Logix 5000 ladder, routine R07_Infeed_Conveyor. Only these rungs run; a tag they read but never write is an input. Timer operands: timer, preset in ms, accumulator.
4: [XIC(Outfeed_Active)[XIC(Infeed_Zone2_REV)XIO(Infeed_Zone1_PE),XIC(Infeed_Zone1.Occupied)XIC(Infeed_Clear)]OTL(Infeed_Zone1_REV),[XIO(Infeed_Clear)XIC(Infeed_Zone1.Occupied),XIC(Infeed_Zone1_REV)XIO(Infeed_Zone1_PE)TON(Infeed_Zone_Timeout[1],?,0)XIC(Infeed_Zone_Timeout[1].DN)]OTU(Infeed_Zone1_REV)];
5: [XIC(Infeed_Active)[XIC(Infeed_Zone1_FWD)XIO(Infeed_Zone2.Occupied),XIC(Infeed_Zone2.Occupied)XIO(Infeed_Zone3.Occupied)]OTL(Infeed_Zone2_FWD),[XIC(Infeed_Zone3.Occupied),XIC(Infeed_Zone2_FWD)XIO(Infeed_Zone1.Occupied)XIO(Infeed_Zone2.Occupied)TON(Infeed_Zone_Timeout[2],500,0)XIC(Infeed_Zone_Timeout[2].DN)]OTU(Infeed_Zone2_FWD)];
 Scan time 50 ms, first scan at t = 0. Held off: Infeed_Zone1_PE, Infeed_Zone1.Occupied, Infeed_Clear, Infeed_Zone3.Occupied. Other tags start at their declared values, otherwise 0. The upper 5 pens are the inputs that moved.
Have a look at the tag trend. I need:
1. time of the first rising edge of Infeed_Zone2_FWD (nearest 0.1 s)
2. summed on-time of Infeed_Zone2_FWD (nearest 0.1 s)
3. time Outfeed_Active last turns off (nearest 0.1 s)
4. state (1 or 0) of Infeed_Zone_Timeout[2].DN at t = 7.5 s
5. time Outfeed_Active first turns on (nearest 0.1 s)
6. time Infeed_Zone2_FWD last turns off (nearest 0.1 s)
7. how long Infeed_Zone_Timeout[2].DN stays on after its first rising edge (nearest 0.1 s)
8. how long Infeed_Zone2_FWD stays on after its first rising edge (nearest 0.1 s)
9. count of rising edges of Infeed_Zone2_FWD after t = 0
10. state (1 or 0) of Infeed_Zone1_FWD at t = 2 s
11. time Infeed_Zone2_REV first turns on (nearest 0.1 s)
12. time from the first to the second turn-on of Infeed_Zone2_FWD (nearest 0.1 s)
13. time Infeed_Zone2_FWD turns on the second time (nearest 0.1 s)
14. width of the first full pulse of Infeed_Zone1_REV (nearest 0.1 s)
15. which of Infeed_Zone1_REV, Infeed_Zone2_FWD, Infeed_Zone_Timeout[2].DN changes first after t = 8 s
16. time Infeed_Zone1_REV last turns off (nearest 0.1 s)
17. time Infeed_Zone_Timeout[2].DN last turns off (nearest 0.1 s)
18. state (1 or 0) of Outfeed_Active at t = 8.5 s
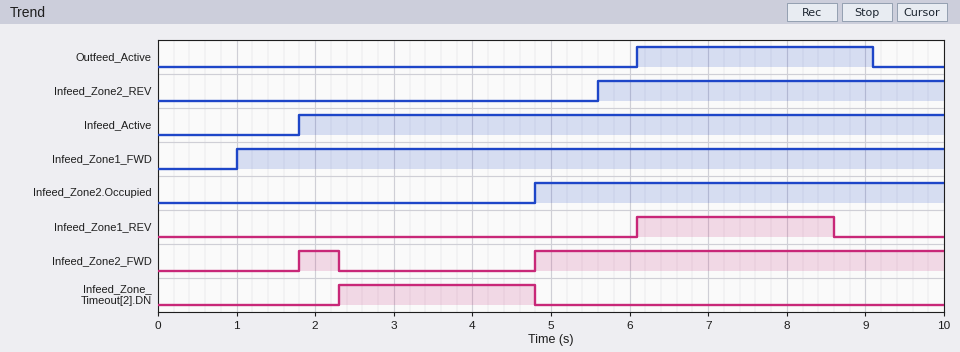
1.8 s
5.7 s
9.1 s
0
6.1 s
2.3 s
2.5 s
0.5 s
2
1
5.6 s
3.0 s
4.8 s
2.5 s
Infeed_Zone1_REV
8.6 s
4.8 s
1
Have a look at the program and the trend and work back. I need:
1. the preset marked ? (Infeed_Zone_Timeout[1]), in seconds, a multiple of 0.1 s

2.5 s
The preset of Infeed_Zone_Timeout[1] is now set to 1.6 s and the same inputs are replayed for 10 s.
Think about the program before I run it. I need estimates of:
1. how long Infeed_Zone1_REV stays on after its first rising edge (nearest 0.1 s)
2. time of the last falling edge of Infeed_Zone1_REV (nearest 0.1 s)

1.6 s
7.7 s
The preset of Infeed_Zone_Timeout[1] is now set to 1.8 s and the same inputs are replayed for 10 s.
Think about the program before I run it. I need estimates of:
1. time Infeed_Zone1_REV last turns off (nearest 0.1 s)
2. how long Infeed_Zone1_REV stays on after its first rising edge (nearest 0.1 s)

7.9 s
1.8 s
